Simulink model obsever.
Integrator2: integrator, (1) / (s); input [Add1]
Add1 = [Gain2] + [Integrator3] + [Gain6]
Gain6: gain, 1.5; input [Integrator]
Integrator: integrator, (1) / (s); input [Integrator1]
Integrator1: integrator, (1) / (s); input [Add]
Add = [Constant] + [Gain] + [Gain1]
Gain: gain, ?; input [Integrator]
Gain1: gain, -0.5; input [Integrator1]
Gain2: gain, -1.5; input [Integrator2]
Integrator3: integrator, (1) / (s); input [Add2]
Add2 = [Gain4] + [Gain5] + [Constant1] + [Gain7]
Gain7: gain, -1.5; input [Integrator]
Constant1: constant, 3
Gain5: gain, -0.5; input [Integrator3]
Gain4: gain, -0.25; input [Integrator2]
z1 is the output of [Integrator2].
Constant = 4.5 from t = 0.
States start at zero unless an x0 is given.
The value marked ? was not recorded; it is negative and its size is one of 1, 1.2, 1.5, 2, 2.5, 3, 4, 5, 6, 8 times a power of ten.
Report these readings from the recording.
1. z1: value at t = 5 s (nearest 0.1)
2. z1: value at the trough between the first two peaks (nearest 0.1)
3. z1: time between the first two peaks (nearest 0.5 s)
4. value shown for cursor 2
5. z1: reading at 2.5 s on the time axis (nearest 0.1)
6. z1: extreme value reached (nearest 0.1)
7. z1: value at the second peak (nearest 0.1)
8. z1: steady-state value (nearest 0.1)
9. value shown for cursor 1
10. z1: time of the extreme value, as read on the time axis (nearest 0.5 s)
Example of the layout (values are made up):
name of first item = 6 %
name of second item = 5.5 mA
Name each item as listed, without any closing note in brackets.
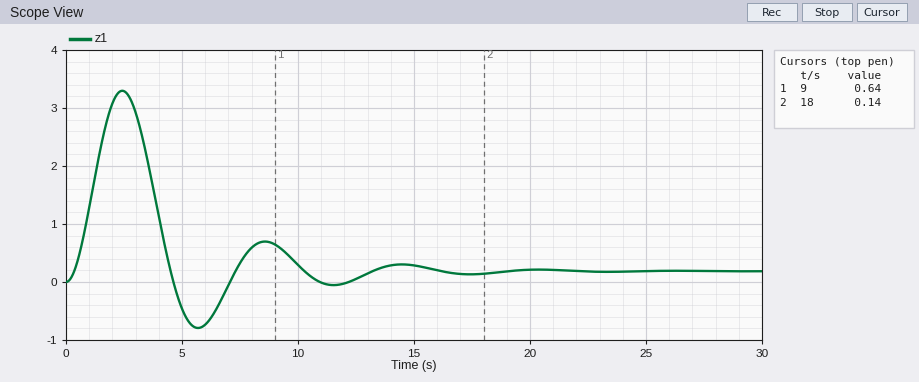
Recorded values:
z1: value at t = 5 s = -0.5
z1: value at the trough between the first two peaks = -0.8
z1: time between the first two peaks = 6.0 s
value shown for cursor 2 = 0.14
z1: reading at 2.5 s on the time axis = 3.3
z1: extreme value reached = 3.3
z1: value at the second peak = 0.7
z1: steady-state value = 0.2
value shown for cursor 1 = 0.64
z1: time of the extreme value, as read on the time axis = 2.5 s
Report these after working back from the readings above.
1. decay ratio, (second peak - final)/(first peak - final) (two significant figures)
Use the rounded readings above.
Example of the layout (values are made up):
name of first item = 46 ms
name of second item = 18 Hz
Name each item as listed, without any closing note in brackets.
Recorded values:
decay ratio, (second peak - final)/(first peak - final) = 0.16
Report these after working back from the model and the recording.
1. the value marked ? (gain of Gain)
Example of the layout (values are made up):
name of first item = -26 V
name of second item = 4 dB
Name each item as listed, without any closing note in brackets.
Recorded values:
the value marked ? = -1.2
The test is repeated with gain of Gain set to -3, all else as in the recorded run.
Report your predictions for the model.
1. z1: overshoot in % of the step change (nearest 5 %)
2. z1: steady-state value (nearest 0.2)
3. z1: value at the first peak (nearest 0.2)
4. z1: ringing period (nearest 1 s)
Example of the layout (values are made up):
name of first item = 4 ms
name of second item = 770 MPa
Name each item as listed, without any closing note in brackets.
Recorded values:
z1: overshoot in % of the step change = 30 %
z1: steady-state value = 1.8
z1: value at the first peak = 2.4
z1: ringing period = 4 s
